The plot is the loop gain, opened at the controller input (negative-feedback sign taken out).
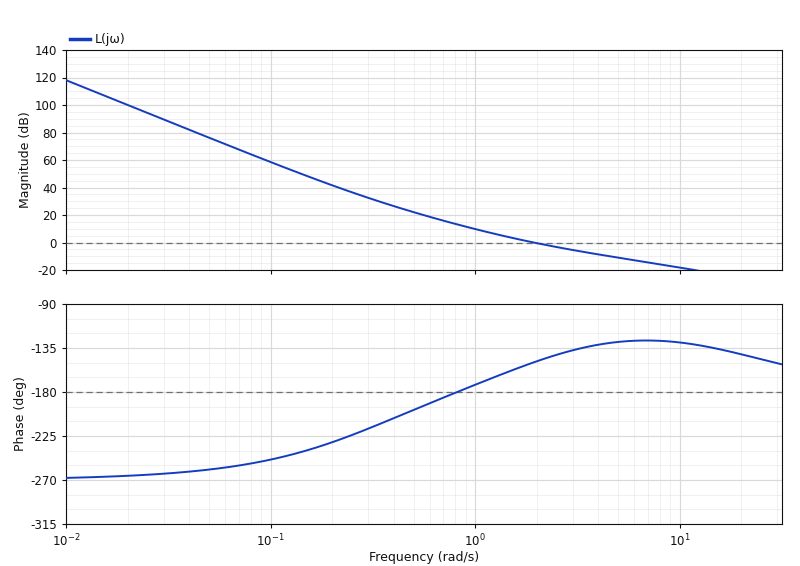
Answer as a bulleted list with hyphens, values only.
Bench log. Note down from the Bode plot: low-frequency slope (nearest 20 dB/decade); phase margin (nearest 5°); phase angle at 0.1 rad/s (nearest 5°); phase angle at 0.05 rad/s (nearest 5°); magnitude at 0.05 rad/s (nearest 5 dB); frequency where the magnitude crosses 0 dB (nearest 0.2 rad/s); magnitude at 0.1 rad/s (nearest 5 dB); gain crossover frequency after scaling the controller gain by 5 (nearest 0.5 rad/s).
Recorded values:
- -60 dB/decade
- 30°
- -250°
- -260°
- 75 dB
- 2.0 rad/s
- 60 dB
- 6.5 rad/s
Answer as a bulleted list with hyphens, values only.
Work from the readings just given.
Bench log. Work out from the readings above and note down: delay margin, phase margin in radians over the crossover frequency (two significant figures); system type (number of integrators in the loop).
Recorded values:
- 0.26 s
- 3
